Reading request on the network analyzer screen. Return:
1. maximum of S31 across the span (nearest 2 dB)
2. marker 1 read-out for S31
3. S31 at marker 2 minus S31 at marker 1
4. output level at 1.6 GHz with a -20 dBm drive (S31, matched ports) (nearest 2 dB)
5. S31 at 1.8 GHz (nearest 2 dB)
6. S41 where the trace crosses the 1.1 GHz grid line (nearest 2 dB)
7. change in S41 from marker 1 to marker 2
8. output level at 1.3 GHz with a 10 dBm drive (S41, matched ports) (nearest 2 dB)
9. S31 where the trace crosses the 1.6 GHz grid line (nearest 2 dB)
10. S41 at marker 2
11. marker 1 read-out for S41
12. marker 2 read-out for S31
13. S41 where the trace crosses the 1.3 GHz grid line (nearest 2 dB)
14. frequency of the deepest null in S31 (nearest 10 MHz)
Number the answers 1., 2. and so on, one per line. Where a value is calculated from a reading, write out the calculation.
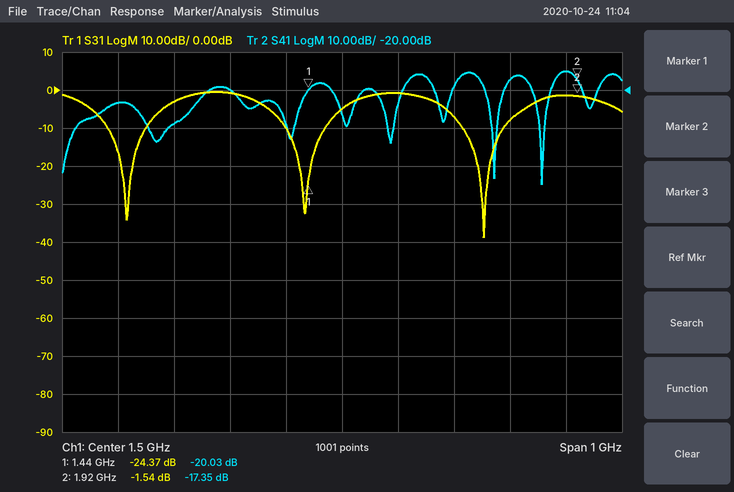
1. 0 dB
2. -24.37 dB
3. -1.54 − (-24.37) = 22.83 dB
4. -20 dBm + (0 dB) = -20 dBm
5. -8 dB
6. -24 dB
7. -17.35 − (-20.03) = 2.68 dB
8. 10 dBm + (-20 dB) = -10 dBm
9. 0 dB
10. -17.35 dB
11. -20.03 dB
12. -1.54 dB
13. -20 dB
14. 1.75 GHz
